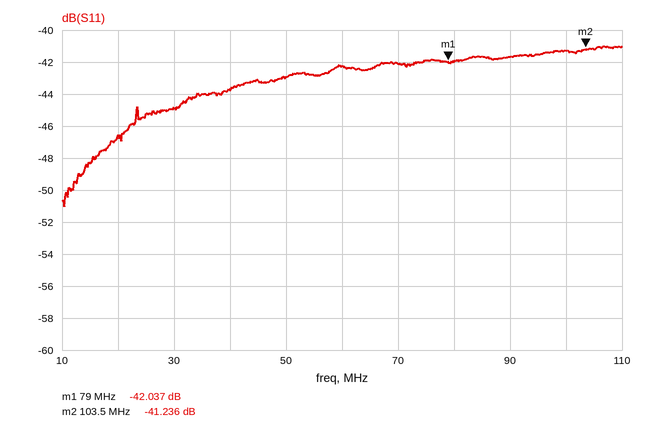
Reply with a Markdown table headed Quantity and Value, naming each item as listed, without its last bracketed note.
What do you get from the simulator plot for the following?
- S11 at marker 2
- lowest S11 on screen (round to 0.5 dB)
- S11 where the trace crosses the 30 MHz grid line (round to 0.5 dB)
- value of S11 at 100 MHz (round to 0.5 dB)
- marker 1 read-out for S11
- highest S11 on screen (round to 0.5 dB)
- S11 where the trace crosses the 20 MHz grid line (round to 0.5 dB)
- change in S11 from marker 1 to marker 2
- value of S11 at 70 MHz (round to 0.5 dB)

| Quantity | Value |
|---|---|
| S11 at marker 2 | -41.236 dB |
| lowest S11 on screen | -51.0 dB |
| S11 where the trace crosses the 30 MHz grid line | -45.0 dB |
| value of S11 at 100 MHz | -41.5 dB |
| marker 1 read-out for S11 | -42.037 dB |
| highest S11 on screen | -41.0 dB |
| S11 where the trace crosses the 20 MHz grid line | -46.5 dB |
| change in S11 from marker 1 to marker 2 | 0.801 dB |
| value of S11 at 70 MHz | -42.0 dB |
